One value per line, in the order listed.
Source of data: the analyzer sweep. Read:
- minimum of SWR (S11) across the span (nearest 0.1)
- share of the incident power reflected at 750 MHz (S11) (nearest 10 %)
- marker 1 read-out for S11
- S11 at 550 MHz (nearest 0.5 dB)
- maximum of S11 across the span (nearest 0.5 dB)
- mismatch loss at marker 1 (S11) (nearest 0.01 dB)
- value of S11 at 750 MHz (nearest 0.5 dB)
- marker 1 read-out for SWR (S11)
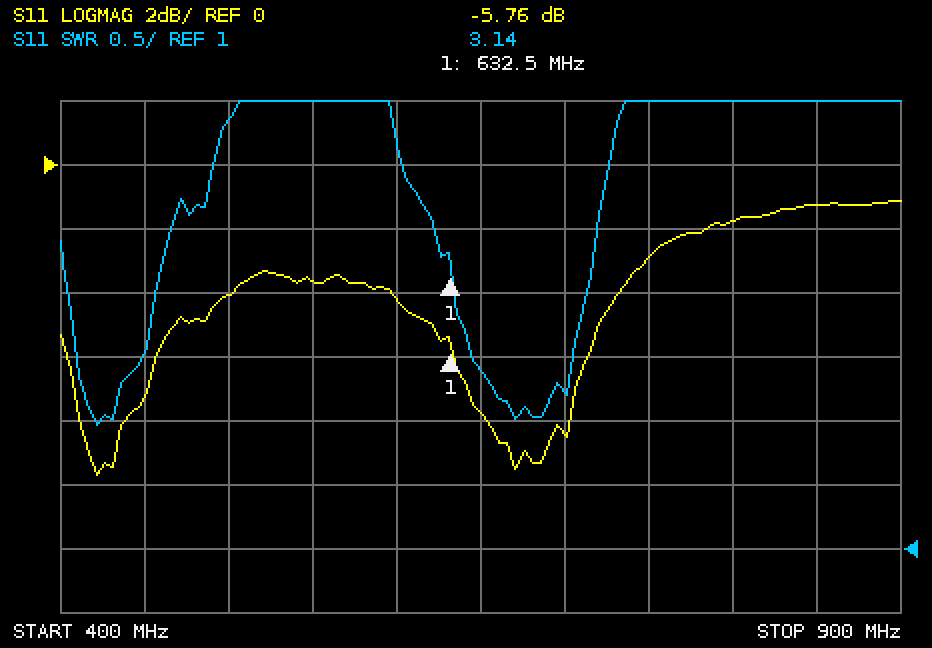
2.0
50 %
-5.76 dB
-3.5 dB
-1.0 dB
1.34 dB
-3.0 dB
3.14
